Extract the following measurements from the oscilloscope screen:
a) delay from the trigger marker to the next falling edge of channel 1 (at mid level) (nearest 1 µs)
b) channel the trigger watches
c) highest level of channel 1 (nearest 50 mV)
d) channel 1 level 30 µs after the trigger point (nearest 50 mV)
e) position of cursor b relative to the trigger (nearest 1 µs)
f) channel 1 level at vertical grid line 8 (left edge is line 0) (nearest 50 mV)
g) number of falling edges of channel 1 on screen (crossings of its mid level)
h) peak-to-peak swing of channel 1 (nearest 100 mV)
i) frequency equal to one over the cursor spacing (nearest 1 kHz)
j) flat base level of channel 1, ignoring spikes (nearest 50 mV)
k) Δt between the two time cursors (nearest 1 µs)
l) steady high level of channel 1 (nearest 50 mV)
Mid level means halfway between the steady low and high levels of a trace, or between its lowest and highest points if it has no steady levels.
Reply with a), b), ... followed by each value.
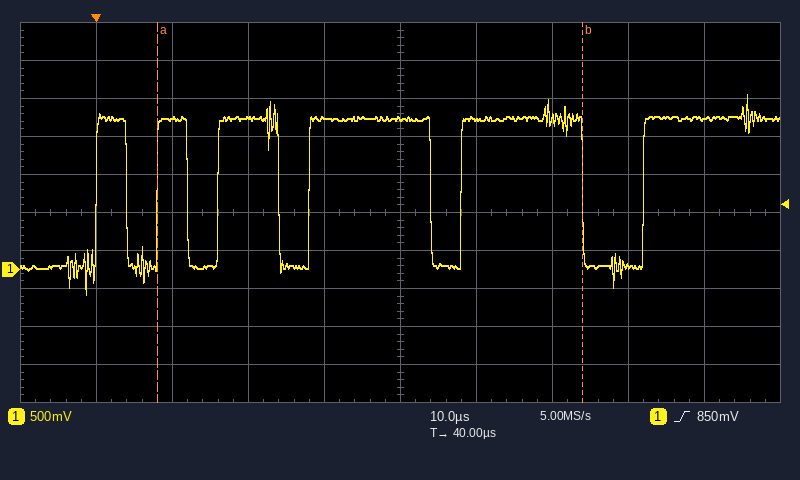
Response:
a) 4 µs
b) channel 1
c) 2.30 V
d) 2.00 V
e) +64 µs
f) 50 mV
g) 5
h) 2.60 V
i) 18 kHz
j) 50 mV
k) 56 µs
l) 2.00 V
